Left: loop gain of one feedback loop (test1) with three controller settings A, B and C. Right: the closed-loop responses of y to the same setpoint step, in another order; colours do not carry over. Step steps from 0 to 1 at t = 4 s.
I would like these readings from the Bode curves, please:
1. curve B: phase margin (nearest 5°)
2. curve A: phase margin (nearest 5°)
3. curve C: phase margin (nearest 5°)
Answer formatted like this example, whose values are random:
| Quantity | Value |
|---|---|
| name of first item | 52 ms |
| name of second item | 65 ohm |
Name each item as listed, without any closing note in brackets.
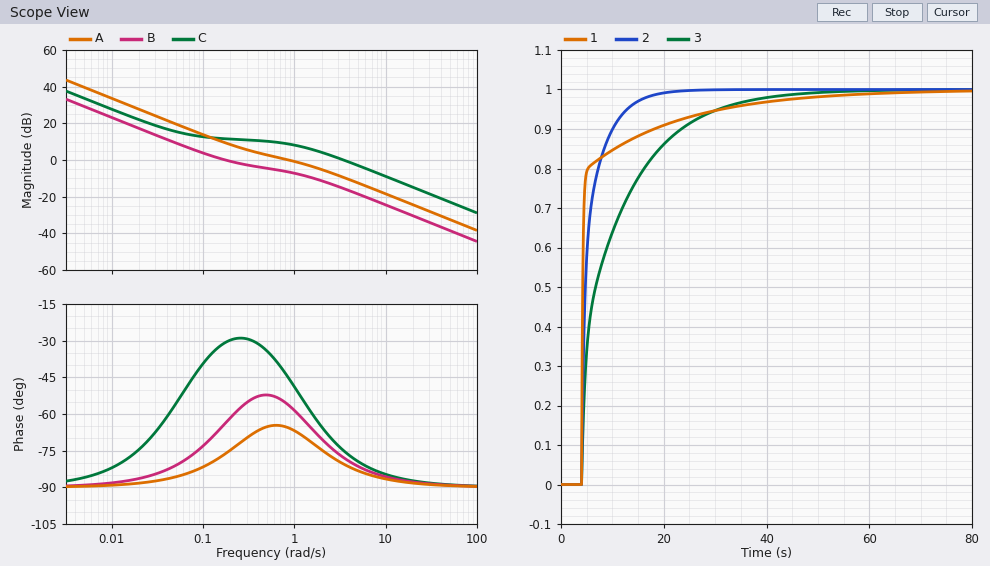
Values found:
| Quantity | Value |
|---|---|
| curve B: phase margin | 115° |
| curve A: phase margin | 115° |
| curve C: phase margin | 105° |
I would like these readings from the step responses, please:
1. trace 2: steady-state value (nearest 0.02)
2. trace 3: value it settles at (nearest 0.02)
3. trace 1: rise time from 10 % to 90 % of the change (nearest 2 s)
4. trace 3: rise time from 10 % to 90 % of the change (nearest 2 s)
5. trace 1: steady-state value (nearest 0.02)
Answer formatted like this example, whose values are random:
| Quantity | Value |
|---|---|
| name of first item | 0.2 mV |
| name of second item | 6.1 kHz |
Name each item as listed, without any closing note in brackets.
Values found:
| Quantity | Value |
|---|---|
| trace 2: steady-state value | 1.00 |
| trace 3: value it settles at | 1.00 |
| trace 1: rise time from 10 % to 90 % of the change | 14 s |
| trace 3: rise time from 10 % to 90 % of the change | 20 s |
| trace 1: steady-state value | 1.00 |
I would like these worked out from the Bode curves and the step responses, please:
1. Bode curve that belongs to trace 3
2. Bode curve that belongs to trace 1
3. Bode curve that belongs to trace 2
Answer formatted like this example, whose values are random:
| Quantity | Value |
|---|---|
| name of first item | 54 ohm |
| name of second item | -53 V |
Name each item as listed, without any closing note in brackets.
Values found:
| Quantity | Value |
|---|---|
| Bode curve that belongs to trace 3 | B |
| Bode curve that belongs to trace 1 | C |
| Bode curve that belongs to trace 2 | A |
